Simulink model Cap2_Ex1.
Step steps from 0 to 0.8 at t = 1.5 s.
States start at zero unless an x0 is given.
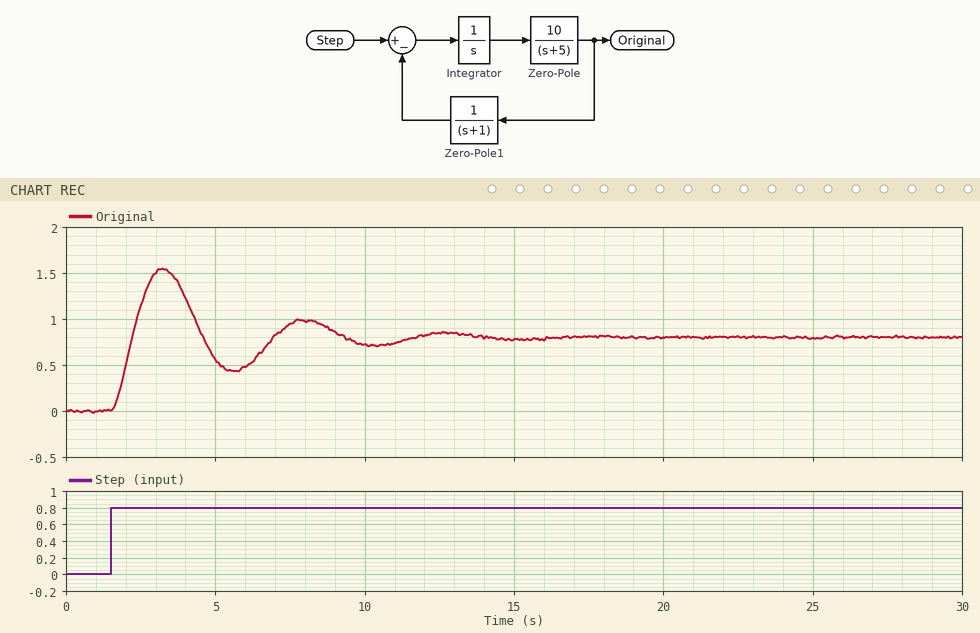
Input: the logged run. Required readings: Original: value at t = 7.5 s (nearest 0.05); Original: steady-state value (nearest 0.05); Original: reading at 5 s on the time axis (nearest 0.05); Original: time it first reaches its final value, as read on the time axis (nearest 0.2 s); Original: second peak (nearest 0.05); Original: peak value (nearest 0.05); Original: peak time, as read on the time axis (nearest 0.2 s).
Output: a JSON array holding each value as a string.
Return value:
["0.95", "0.80", "0.55", "2.2 s", "1.00", "1.55", "3.2 s"]
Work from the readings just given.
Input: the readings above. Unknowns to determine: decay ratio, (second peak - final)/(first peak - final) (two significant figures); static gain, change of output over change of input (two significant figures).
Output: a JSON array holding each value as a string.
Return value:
["0.27", "1.0"]
